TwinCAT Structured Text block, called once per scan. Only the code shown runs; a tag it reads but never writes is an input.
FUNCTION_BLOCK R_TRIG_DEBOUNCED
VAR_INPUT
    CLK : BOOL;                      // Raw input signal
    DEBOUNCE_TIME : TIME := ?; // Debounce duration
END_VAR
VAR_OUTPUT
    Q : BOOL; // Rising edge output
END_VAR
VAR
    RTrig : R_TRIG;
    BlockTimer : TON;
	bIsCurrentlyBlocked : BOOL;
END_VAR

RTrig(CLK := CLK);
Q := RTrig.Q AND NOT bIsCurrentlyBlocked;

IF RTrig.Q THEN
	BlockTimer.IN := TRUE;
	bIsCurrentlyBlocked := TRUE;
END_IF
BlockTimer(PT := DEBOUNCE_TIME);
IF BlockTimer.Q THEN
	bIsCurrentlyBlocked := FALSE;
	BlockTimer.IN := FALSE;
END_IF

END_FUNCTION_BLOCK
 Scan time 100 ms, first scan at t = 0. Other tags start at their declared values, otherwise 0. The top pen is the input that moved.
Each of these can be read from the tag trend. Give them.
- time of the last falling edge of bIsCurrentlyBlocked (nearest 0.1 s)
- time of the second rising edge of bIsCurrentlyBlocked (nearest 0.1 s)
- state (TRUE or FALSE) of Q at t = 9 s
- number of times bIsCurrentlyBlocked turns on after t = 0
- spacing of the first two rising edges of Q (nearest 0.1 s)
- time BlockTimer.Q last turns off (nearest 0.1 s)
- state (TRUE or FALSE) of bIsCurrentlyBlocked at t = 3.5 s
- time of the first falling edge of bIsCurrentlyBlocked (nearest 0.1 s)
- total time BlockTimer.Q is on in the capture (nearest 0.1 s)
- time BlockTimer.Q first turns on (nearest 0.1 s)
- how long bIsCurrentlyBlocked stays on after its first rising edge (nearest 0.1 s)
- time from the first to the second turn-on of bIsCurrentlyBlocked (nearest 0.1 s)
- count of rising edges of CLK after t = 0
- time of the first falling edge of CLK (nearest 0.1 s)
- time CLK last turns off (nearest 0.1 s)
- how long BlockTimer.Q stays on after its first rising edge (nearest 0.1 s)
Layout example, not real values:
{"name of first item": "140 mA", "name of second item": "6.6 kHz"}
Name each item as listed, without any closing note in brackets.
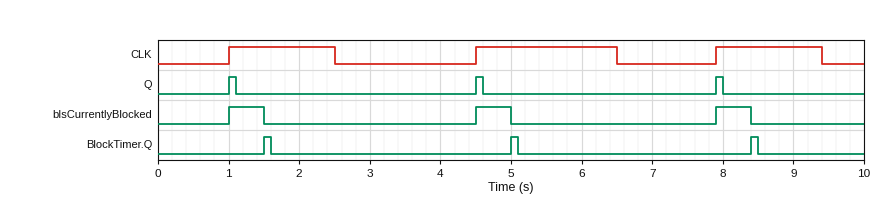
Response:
{"time of the last falling edge of bIsCurrentlyBlocked": "8.4 s", "time of the second rising edge of bIsCurrentlyBlocked": "4.5 s", "state (TRUE or FALSE) of Q at t = 9 s": "FALSE", "number of times bIsCurrentlyBlocked turns on after t = 0": "3", "spacing of the first two rising edges of Q": "3.5 s", "time BlockTimer.Q last turns off": "8.5 s", "state (TRUE or FALSE) of bIsCurrentlyBlocked at t = 3.5 s": "FALSE", "time of the first falling edge of bIsCurrentlyBlocked": "1.5 s", "total time BlockTimer.Q is on in the capture": "0.3 s", "time BlockTimer.Q first turns on": "1.5 s", "how long bIsCurrentlyBlocked stays on after its first rising edge": "0.5 s", "time from the first to the second turn-on of bIsCurrentlyBlocked": "3.5 s", "count of rising edges of CLK after t = 0": "3", "time of the first falling edge of CLK": "2.5 s", "time CLK last turns off": "9.4 s", "how long BlockTimer.Q stays on after its first rising edge": "0.1 s"}
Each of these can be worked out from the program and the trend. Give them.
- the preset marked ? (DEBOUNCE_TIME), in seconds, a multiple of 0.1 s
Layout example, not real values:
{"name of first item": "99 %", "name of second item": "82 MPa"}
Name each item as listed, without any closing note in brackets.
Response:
{"the preset marked ? (DEBOUNCE_TIME), in seconds, a multiple of 0.1 s": "0.5 s"}
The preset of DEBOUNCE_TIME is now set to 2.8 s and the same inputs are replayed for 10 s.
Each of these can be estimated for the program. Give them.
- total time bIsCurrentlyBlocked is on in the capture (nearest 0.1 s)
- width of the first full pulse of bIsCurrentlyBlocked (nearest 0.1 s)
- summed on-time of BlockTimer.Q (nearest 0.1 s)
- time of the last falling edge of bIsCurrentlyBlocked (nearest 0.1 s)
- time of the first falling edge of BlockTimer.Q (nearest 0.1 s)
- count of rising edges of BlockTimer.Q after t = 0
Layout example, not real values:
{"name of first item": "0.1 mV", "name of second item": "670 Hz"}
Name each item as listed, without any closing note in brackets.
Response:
{"total time bIsCurrentlyBlocked is on in the capture": "7.7 s", "width of the first full pulse of bIsCurrentlyBlocked": "2.8 s", "summed on-time of BlockTimer.Q": "0.2 s", "time of the last falling edge of bIsCurrentlyBlocked": "7.3 s", "time of the first falling edge of BlockTimer.Q": "3.9 s", "count of rising edges of BlockTimer.Q after t = 0": "2"}
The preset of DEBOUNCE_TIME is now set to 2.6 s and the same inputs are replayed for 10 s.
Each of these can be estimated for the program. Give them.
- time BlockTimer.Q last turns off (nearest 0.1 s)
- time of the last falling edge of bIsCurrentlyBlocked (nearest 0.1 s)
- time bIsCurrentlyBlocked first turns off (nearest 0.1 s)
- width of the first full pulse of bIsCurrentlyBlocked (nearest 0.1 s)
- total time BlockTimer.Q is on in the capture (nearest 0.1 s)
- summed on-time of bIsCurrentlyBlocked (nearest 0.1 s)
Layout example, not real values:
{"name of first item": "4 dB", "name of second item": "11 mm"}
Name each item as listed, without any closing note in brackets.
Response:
{"time BlockTimer.Q last turns off": "7.2 s", "time of the last falling edge of bIsCurrentlyBlocked": "7.1 s", "time bIsCurrentlyBlocked first turns off": "3.6 s", "width of the first full pulse of bIsCurrentlyBlocked": "2.6 s", "total time BlockTimer.Q is on in the capture": "0.2 s", "summed on-time of bIsCurrentlyBlocked": "7.3 s"}
